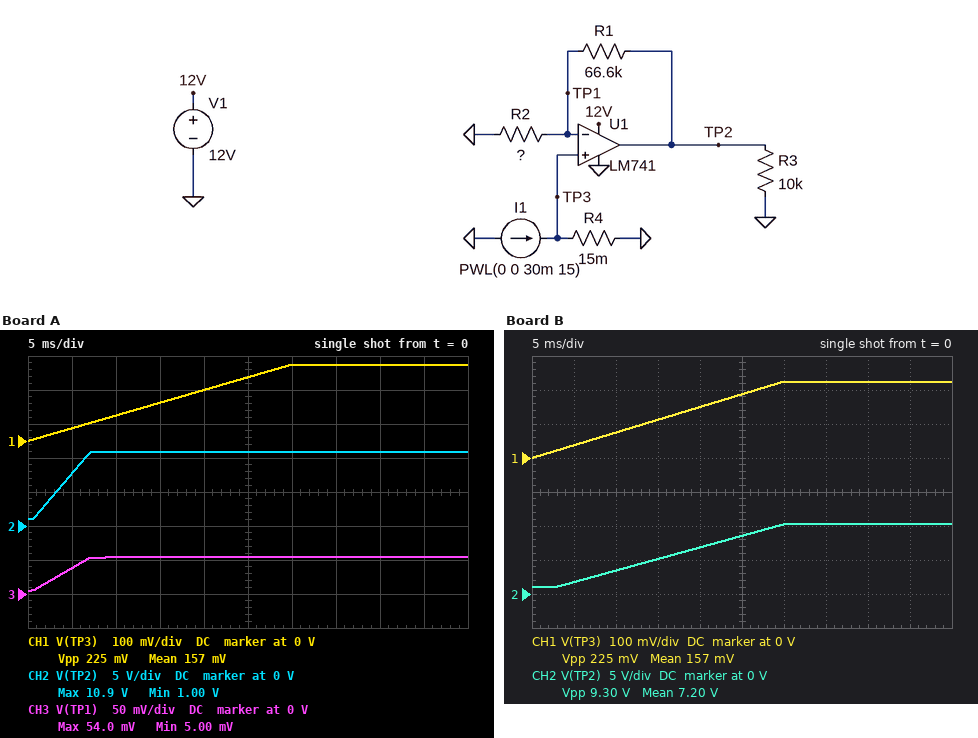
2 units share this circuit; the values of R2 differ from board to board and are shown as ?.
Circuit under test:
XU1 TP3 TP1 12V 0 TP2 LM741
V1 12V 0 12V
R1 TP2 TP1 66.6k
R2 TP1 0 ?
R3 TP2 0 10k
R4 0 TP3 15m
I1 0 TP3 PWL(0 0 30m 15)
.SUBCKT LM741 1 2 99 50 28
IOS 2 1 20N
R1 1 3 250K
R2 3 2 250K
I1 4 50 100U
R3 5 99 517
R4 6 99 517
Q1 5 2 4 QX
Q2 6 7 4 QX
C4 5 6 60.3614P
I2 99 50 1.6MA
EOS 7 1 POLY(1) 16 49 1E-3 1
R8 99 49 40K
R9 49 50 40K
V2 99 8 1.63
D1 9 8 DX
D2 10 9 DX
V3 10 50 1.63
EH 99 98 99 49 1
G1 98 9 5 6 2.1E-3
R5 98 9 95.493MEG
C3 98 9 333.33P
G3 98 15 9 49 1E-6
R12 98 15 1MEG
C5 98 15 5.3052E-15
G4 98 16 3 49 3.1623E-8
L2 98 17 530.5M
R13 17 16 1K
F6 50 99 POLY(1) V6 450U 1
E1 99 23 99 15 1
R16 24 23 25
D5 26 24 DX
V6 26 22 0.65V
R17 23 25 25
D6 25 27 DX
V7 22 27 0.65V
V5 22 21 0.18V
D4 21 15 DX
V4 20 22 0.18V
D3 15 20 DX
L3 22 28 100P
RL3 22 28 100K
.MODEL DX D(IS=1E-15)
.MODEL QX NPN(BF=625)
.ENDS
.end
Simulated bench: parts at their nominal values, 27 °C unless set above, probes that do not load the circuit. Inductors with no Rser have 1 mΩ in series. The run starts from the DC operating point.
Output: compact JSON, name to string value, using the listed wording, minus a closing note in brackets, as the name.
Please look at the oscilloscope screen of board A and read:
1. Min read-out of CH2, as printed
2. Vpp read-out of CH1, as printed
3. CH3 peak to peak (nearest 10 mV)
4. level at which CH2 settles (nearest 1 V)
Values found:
{"Min read-out of CH2, as printed": "1.00 V", "Vpp read-out of CH1, as printed": "225 mV", "CH3 peak to peak": "50 mV", "level at which CH2 settles": "11 V"}
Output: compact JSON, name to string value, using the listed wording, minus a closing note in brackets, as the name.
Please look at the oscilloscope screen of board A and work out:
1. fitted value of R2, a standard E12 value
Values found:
{"fitted value of R2, a standard E12 value": "330 Ω"}
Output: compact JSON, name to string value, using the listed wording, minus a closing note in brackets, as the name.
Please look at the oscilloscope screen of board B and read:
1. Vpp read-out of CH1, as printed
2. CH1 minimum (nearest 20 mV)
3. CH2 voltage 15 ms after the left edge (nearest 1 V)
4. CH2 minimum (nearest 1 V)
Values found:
{"Vpp read-out of CH1, as printed": "225 mV", "CH1 minimum": "0 V", "CH2 voltage 15 ms after the left edge": "5 V", "CH2 minimum": "1 V"}
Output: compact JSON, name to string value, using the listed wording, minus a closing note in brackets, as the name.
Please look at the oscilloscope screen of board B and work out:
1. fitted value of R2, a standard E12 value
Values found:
{"fitted value of R2, a standard E12 value": "1.5 kΩ"}
